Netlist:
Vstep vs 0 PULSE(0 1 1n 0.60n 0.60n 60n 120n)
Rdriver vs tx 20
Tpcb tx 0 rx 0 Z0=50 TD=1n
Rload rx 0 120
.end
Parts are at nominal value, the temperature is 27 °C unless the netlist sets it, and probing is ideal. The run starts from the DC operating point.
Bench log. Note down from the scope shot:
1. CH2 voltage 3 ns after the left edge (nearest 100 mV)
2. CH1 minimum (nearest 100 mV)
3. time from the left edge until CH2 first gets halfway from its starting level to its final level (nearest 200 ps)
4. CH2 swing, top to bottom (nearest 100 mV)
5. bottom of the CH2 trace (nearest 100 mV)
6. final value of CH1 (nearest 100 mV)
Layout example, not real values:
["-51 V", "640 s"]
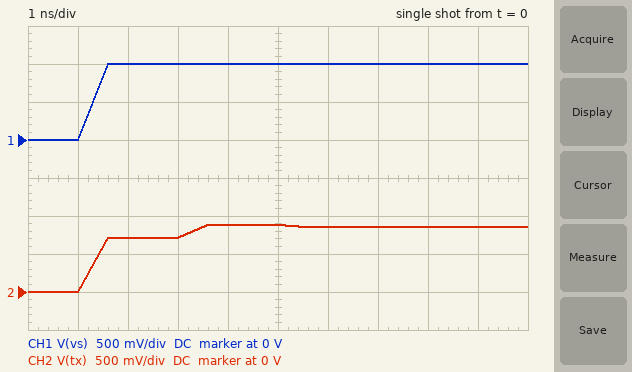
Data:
["700 mV", "0 V", "1.4 ns", "900 mV", "0 V", "1.0 V"]
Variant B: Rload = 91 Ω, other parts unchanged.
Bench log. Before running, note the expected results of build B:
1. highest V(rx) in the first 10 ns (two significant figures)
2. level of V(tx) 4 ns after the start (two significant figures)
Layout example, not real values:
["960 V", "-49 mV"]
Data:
["920 mV", "830 mV"]
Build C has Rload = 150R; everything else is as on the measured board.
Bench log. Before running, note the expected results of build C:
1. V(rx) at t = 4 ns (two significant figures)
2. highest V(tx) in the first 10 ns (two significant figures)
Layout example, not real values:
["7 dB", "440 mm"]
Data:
["1.1 V", "920 mV"]
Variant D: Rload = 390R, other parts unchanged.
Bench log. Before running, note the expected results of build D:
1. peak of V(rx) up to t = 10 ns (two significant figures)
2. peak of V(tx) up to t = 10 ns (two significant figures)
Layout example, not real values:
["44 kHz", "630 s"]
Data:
["1.3 V", "1.0 V"]
